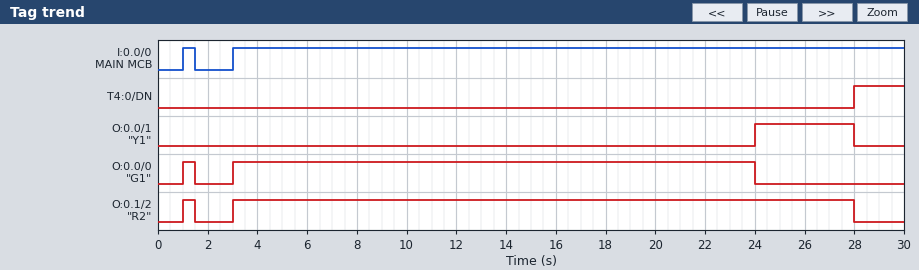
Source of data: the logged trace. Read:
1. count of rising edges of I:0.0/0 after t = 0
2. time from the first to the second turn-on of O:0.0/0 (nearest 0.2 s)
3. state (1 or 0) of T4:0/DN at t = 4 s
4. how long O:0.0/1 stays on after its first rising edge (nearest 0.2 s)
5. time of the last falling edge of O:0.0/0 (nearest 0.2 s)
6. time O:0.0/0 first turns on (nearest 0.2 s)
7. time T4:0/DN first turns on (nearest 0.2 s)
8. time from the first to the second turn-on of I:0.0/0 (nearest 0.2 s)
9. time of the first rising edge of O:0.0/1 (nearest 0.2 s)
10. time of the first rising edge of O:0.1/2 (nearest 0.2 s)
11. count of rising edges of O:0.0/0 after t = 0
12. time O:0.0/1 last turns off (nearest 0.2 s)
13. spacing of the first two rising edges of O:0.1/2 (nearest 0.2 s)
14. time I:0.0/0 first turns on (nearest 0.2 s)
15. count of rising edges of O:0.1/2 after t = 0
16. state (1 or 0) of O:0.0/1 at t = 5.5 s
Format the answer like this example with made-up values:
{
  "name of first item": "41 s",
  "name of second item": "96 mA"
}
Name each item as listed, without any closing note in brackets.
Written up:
{
  "count of rising edges of I:0.0/0 after t = 0": "2",
  "time from the first to the second turn-on of O:0.0/0": "2.0 s",
  "state (1 or 0) of T4:0/DN at t = 4 s": "0",
  "how long O:0.0/1 stays on after its first rising edge": "4.0 s",
  "time of the last falling edge of O:0.0/0": "24.0 s",
  "time O:0.0/0 first turns on": "1.0 s",
  "time T4:0/DN first turns on": "28.0 s",
  "time from the first to the second turn-on of I:0.0/0": "2.0 s",
  "time of the first rising edge of O:0.0/1": "24.0 s",
  "time of the first rising edge of O:0.1/2": "1.0 s",
  "count of rising edges of O:0.0/0 after t = 0": "2",
  "time O:0.0/1 last turns off": "28.0 s",
  "spacing of the first two rising edges of O:0.1/2": "2.0 s",
  "time I:0.0/0 first turns on": "1.0 s",
  "count of rising edges of O:0.1/2 after t = 0": "2",
  "state (1 or 0) of O:0.0/1 at t = 5.5 s": "0"
}
